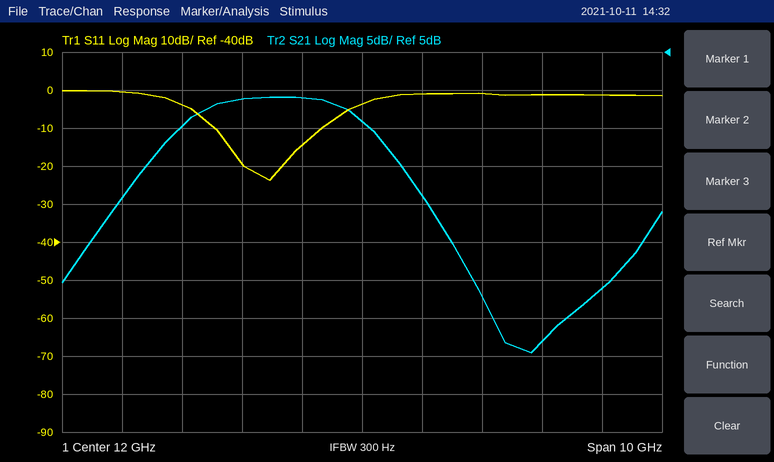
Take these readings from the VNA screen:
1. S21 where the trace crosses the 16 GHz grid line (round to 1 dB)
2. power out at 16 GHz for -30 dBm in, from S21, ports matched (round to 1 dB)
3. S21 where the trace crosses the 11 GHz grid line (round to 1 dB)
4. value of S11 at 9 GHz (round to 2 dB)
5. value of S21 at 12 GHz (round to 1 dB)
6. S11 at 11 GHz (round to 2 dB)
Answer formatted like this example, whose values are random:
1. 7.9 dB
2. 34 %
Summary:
1. -26 dB
2. -56 dBm
3. -1 dB
4. -4 dB
5. -4 dB
6. -14 dB
